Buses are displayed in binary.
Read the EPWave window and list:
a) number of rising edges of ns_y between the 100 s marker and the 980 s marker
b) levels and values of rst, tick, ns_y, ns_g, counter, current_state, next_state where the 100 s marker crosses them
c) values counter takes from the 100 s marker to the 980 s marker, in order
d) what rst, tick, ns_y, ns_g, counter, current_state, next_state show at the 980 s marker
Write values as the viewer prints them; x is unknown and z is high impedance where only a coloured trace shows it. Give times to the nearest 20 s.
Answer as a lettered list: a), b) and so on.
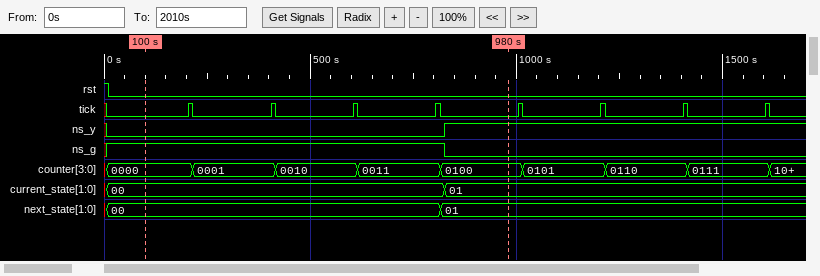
a) 1
b) rst=0, tick=0, ns_y=0, ns_g=1, counter=0000, current_state=00, next_state=00
c) 0000, 0001, 0010, 0011, 0100
d) rst=0, tick=0, ns_y=1, ns_g=0, counter=0100, current_state=01, next_state=01
